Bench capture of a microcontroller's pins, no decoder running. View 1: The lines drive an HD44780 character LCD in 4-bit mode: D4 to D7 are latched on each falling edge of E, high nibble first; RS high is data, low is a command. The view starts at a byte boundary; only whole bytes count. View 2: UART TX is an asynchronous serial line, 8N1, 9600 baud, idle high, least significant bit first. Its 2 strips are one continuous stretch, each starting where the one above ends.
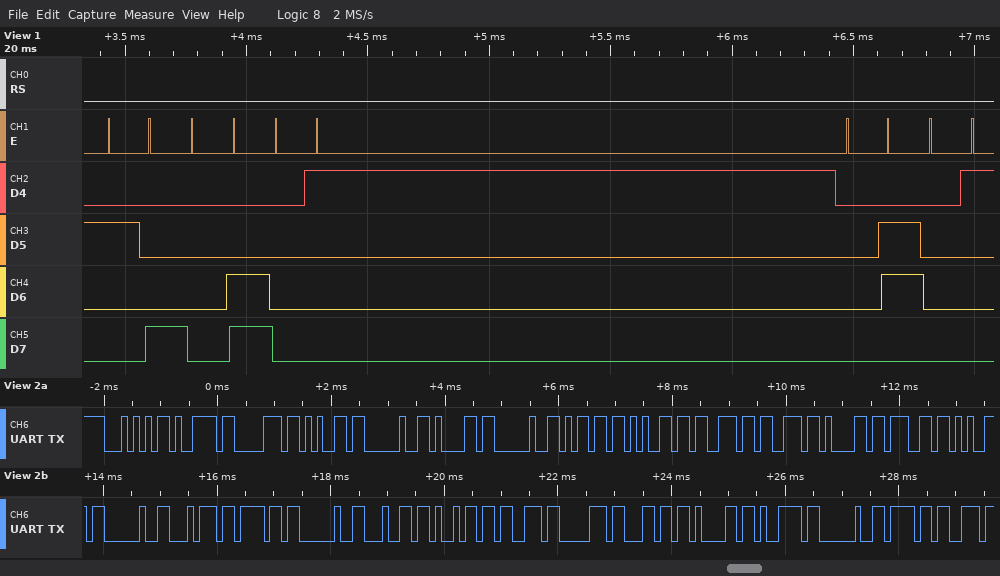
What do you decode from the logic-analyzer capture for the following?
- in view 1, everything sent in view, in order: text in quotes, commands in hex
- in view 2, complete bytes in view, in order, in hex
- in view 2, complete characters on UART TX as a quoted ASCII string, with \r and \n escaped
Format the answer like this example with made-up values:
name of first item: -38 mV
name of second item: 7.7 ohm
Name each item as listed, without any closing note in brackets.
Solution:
in view 1, everything sent in view, in order: text in quotes, commands in hex: 0x28 0x0C 0x01 0x06 0x01
in view 2, complete bytes in view, in order, in hex: 0x54 0x79 0x70 0x65 0x20 0x61 0x20 0x6D 0x65 0x73 0x73 0x61 0x67 0x65 0x20 0x74 0x6F 0x20 0x64 0x69 0x73 0x70 0x6C 0x61 0x79 0x20 0x6F
in view 2, complete characters on UART TX as a quoted ASCII string, with \r and \n escaped: "Type a message to display o"
